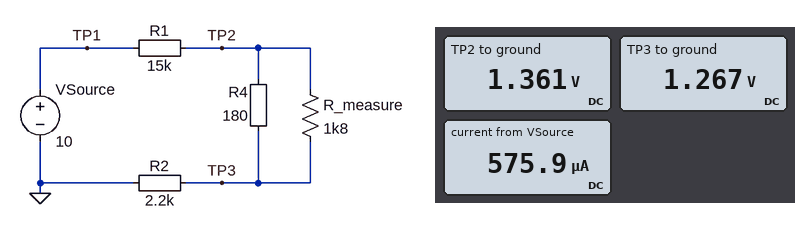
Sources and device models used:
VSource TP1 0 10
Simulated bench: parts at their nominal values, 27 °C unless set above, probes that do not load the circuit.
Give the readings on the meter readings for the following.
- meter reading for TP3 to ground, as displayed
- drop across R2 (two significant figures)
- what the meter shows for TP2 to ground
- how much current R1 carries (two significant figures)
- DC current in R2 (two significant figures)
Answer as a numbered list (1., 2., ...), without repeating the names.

1. 1.267 V
2. 1.3 V
3. 1.361 V
4. 580 µA
5. 580 µA
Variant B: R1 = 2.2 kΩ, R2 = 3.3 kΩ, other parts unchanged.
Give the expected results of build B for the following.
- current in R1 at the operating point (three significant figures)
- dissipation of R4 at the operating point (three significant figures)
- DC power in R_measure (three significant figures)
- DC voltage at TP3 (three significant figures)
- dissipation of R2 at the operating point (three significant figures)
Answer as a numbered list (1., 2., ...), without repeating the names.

1. 1.77 mA
2. 464 µW
3. 46.4 µW
4. 5.83 V
5. 10.3 mW
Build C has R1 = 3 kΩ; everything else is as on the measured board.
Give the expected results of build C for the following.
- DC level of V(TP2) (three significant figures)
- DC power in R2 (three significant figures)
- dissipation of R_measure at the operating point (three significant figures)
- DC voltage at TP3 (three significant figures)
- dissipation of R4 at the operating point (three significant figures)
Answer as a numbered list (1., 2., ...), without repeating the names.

1. 4.41 V
2. 7.65 mW
3. 51.7 µW
4. 4.10 V
5. 517 µW
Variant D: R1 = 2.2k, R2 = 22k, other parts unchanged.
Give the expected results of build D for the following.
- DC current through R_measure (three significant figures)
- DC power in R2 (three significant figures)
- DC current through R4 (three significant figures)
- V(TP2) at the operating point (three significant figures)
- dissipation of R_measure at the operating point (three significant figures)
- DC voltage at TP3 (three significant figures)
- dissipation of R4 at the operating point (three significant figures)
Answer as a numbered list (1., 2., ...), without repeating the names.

1. 37.3 µA
2. 3.71 mW
3. 373 µA
4. 9.10 V
5. 2.51 µW
6. 9.03 V
7. 25.1 µW
